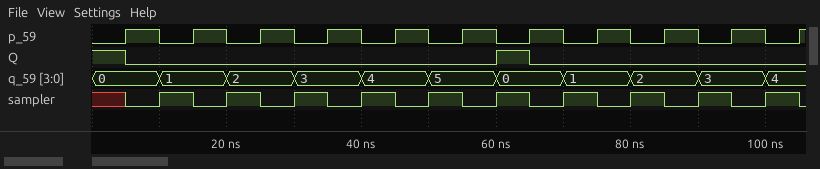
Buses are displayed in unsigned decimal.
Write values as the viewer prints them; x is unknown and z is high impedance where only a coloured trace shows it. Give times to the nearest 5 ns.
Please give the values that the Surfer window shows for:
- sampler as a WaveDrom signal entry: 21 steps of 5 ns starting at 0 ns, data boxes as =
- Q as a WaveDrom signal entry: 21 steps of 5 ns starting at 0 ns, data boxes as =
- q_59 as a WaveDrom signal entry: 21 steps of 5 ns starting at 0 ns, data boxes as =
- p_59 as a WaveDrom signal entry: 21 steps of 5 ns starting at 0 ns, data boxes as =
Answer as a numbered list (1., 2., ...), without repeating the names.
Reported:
1. {name: 'sampler', wave: 'x01010101010101010101'}
2. {name: 'Q', wave: '10..........10.......'}
3. {name: 'q_59', wave: '=.=.=.=.=.=.=.=.=.=.=', data: '0 1 2 3 4 5 0 1 2 3 4'}
4. {name: 'p_59', wave: '010101010101010101010'}
